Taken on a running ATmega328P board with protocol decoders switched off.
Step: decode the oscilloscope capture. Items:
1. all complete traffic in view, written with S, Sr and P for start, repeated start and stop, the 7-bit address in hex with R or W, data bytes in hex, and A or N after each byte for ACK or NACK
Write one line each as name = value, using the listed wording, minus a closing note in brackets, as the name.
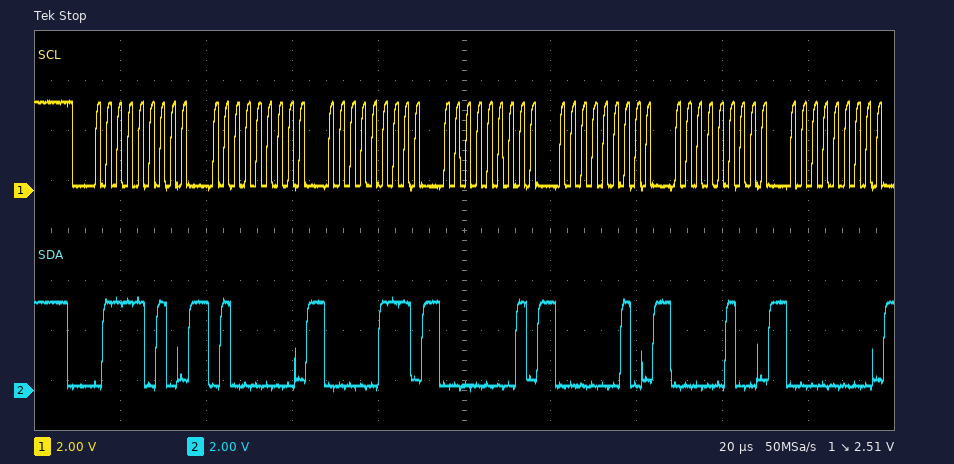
all complete traffic in view, written with S, Sr and P for start, repeated start and stop, the 7-bit address in hex with R or W, data bytes in hex, and A or N after each byte for ACK or NACK = S 3DW A 40 A 07 A 01 A 02 A 04 A 00 A
